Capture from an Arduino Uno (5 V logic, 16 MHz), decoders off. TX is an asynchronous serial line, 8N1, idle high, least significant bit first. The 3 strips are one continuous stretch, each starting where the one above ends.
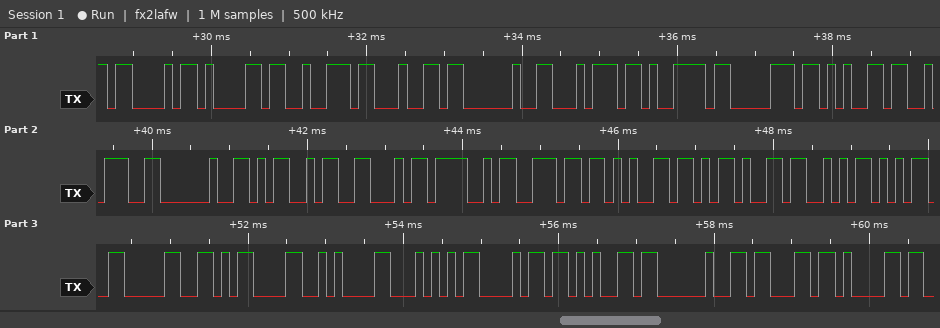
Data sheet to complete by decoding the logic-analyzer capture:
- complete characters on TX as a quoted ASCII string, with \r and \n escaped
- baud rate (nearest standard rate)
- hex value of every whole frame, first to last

"Card type: MFOne-S50\r\nThe ca"
9600 baud
43 61 72 64 20 74 79 70 65 3A 20 4D 46 4F 6E 65 2D 53 35 30 0D 0A 54 68 65 20 63 61
